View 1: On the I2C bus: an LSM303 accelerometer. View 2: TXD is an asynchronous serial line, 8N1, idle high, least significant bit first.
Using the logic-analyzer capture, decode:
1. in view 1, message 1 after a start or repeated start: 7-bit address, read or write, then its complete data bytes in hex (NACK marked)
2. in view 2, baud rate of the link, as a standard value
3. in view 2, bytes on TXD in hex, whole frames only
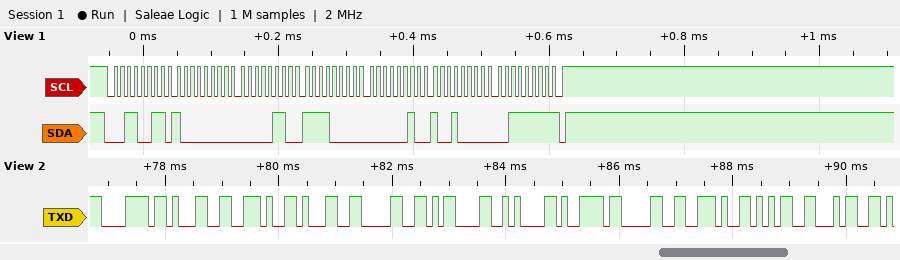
0x19 read: 80 06 F0 02 90 3F NACK
9600 baud
78 31 2E 31 30 0D 0A 79 30 2E 35 34
